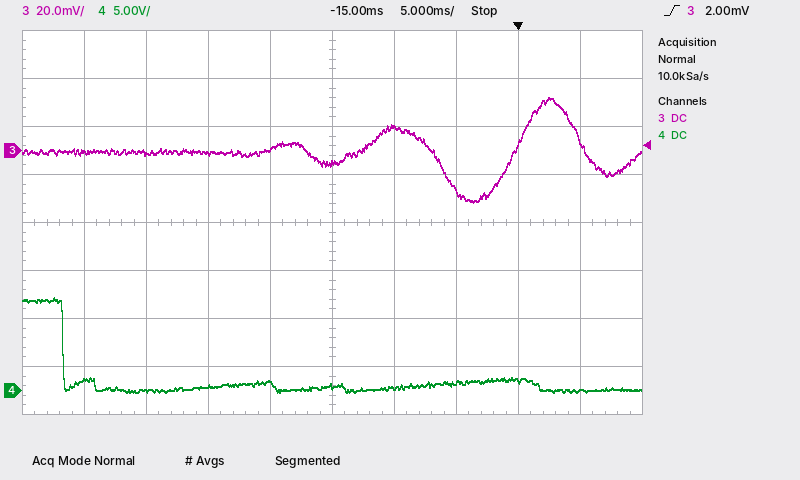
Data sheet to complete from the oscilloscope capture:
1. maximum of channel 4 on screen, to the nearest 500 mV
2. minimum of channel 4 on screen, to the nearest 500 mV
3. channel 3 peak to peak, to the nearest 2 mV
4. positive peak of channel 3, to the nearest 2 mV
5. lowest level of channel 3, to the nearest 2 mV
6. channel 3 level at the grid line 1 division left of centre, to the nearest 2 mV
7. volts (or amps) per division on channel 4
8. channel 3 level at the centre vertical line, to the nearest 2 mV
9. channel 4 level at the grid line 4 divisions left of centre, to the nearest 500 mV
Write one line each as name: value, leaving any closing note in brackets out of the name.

maximum of channel 4 on screen, to the nearest 500 mV: 9.5 V
minimum of channel 4 on screen, to the nearest 500 mV: 0.0 V
channel 3 peak to peak, to the nearest 2 mV: 44 mV
positive peak of channel 3, to the nearest 2 mV: 22 mV
lowest level of channel 3, to the nearest 2 mV: -22 mV
channel 3 level at the grid line 1 division left of centre, to the nearest 2 mV: 0 mV
volts (or amps) per division on channel 4: 5 V
channel 3 level at the centre vertical line, to the nearest 2 mV: -6 mV
channel 4 level at the grid line 4 divisions left of centre, to the nearest 500 mV: 1.0 V
